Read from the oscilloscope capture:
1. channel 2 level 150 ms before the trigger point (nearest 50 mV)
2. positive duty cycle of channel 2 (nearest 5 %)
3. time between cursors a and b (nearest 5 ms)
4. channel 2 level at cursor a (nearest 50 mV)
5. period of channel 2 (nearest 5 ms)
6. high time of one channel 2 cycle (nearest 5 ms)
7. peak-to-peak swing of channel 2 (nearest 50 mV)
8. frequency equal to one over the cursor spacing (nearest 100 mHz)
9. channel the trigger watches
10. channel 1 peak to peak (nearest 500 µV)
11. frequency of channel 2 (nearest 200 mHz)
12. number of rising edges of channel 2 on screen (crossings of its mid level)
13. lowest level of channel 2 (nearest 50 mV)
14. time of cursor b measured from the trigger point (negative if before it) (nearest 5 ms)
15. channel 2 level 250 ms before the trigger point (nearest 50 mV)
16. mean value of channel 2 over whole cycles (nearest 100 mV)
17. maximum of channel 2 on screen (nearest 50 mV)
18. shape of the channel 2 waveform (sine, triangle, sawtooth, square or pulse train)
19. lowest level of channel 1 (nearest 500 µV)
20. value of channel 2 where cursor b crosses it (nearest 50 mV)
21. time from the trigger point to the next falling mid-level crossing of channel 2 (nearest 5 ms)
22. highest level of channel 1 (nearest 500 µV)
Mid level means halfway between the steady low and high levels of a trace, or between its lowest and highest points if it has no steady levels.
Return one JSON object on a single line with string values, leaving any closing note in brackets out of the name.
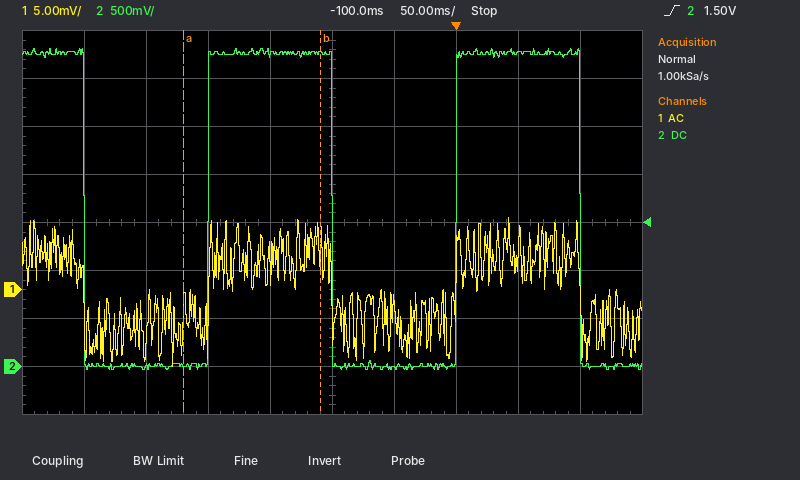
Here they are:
{"channel 2 level 150 ms before the trigger point": "3.25 V", "positive duty cycle of channel 2": "50 %", "time between cursors a and b": "110 ms", "channel 2 level at cursor a": "0 mV", "period of channel 2": "200 ms", "high time of one channel 2 cycle": "100 ms", "peak-to-peak swing of channel 2": "3.35 V", "frequency equal to one over the cursor spacing": "9.1 Hz", "channel the trigger watches": "channel 2", "channel 1 peak to peak": "15.5 mV", "frequency of channel 2": "5.0 Hz", "number of rising edges of channel 2 on screen": "2", "lowest level of channel 2": "-50 mV", "time of cursor b measured from the trigger point (negative if before it)": "-110 ms", "channel 2 level 250 ms before the trigger point": "0 mV", "mean value of channel 2 over whole cycles": "1.6 V", "maximum of channel 2 on screen": "3.30 V", "shape of the channel 2 waveform": "square", "lowest level of channel 1": "-8.0 mV", "value of channel 2 where cursor b crosses it": "3.25 V", "time from the trigger point to the next falling mid-level crossing of channel 2": "100 ms", "highest level of channel 1": "7.5 mV"}
